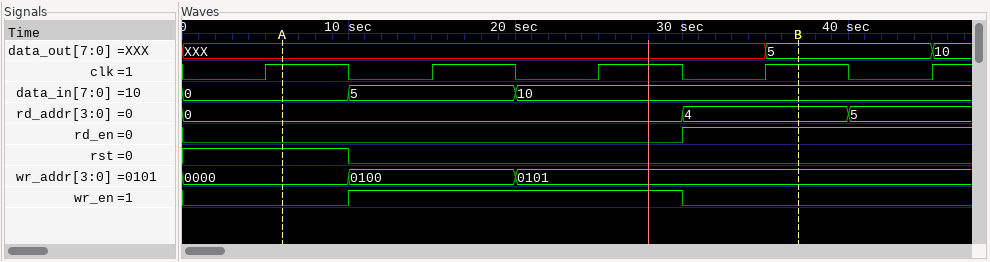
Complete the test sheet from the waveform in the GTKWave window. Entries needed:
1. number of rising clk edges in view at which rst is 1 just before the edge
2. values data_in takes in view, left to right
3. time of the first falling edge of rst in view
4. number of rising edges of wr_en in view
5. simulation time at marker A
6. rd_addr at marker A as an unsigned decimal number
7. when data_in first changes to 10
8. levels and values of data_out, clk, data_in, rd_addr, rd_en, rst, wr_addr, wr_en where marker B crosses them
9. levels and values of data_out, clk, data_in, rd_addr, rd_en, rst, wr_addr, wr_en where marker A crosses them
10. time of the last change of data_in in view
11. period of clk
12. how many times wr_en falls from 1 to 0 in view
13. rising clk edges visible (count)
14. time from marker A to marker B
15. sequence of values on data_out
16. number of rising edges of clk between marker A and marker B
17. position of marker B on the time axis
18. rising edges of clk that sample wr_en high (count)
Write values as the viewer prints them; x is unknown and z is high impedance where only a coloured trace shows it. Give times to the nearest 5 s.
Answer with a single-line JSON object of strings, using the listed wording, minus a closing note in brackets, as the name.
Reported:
{"number of rising clk edges in view at which rst is 1 just before the edge": "1", "values data_in takes in view, left to right": "0, 5, 10", "time of the first falling edge of rst in view": "10 s", "number of rising edges of wr_en in view": "1", "simulation time at marker A": "5 s", "rd_addr at marker A as an unsigned decimal number": "0", "when data_in first changes to 10": "20 s", "levels and values of data_out, clk, data_in, rd_addr, rd_en, rst, wr_addr, wr_en where marker B crosses them": "data_out=5, clk=1, data_in=10, rd_addr=4, rd_en=1, rst=0, wr_addr=0101, wr_en=0", "levels and values of data_out, clk, data_in, rd_addr, rd_en, rst, wr_addr, wr_en where marker A crosses them": "data_out=XXX, clk=1, data_in=0, rd_addr=0, rd_en=0, rst=1, wr_addr=0000, wr_en=0", "time of the last change of data_in in view": "20 s", "period of clk": "10 s", "how many times wr_en falls from 1 to 0 in view": "1", "rising clk edges visible": "5", "time from marker A to marker B": "30 s", "sequence of values on data_out": "XXX, 5, 10", "number of rising edges of clk between marker A and marker B": "3", "position of marker B on the time axis": "35 s", "rising edges of clk that sample wr_en high": "2"}
